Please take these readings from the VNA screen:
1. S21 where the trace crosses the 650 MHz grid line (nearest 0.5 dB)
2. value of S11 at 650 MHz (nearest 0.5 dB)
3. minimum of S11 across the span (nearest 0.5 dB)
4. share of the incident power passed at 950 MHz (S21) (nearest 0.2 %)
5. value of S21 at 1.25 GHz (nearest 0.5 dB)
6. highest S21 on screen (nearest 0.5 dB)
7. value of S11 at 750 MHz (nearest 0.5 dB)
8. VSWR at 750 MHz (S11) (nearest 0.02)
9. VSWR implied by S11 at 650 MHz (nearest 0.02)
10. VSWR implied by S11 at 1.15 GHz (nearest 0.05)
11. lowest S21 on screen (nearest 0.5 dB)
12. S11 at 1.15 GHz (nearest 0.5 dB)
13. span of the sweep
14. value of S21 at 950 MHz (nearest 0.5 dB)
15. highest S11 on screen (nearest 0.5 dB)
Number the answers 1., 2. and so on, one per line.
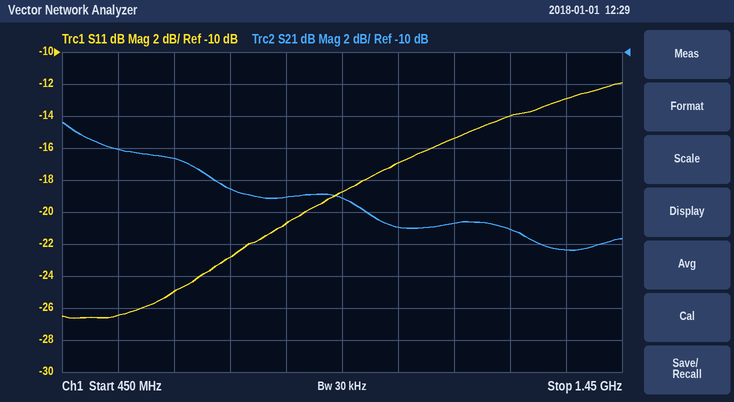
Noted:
1. -16.5 dB
2. -25.0 dB
3. -26.5 dB
4. 1.2 %
5. -21.0 dB
6. -14.5 dB
7. -23.0 dB
8. 1.16
9. 1.12
10. 1.40
11. -22.5 dB
12. -15.5 dB
13. 1 GHz
14. -19.0 dB
15. -12.0 dB
